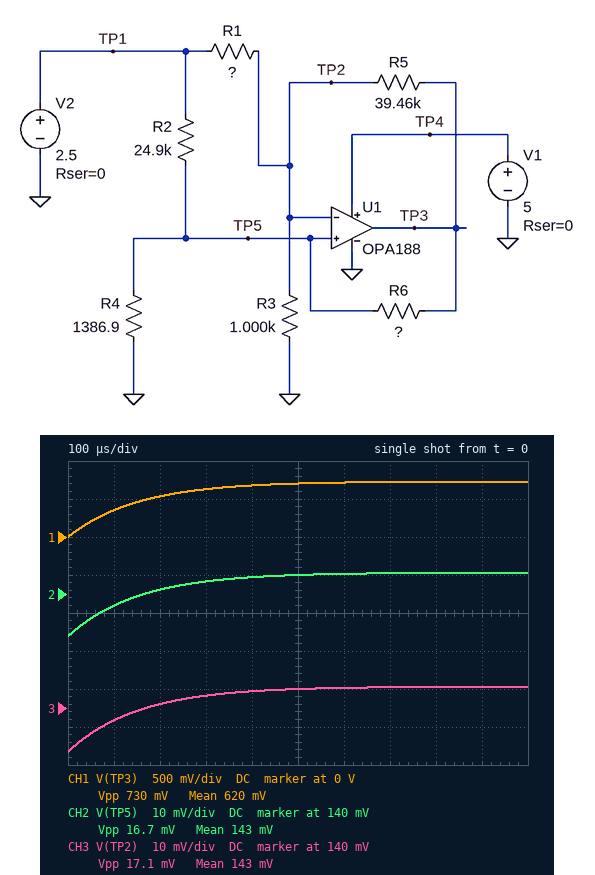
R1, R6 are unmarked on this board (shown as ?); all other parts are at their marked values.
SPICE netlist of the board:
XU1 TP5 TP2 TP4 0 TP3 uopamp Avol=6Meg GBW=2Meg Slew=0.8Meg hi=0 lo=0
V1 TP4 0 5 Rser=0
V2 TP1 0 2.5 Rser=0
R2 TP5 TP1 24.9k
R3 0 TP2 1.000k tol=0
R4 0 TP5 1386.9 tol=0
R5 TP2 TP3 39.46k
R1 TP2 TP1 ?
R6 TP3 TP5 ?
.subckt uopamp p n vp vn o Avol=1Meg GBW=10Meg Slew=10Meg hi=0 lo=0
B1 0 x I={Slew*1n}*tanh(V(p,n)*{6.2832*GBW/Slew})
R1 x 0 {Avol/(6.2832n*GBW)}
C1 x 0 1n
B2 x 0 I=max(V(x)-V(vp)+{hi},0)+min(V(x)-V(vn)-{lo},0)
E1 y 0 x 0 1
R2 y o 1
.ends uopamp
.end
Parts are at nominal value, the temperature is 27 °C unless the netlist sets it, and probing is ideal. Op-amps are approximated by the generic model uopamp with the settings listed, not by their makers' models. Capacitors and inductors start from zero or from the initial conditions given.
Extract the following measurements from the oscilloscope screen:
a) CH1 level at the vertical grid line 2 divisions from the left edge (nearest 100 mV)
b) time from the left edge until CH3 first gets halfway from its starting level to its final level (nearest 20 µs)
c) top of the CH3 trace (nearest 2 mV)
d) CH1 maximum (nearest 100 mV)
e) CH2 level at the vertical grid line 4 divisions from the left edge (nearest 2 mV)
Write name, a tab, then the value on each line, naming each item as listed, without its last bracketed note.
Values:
CH1 level at the vertical grid line 2 divisions from the left edge	500 mV
time from the left edge until CH3 first gets halfway from its starting level to its final level	100 µs
top of the CH3 trace	146 mV
CH1 maximum	700 mV
CH2 level at the vertical grid line 4 divisions from the left edge	144 mV
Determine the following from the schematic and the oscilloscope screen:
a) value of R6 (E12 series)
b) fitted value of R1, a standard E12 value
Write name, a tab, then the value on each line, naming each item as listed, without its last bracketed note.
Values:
value of R6	56 kΩ
fitted value of R1, a standard E12 value	18 kΩ
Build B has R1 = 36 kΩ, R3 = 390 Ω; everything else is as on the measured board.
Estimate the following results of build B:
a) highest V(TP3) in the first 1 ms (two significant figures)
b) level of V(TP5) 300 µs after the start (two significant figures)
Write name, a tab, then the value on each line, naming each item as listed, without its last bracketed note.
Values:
highest V(TP3) in the first 1 ms	5.0 V
level of V(TP5) 300 µs after the start	240 mV
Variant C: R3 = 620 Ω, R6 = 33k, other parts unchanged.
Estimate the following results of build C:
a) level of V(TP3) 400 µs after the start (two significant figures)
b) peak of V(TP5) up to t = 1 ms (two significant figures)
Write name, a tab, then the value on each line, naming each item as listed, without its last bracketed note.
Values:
level of V(TP3) 400 µs after the start	5.0 V
peak of V(TP5) up to t = 1 ms	320 mV
